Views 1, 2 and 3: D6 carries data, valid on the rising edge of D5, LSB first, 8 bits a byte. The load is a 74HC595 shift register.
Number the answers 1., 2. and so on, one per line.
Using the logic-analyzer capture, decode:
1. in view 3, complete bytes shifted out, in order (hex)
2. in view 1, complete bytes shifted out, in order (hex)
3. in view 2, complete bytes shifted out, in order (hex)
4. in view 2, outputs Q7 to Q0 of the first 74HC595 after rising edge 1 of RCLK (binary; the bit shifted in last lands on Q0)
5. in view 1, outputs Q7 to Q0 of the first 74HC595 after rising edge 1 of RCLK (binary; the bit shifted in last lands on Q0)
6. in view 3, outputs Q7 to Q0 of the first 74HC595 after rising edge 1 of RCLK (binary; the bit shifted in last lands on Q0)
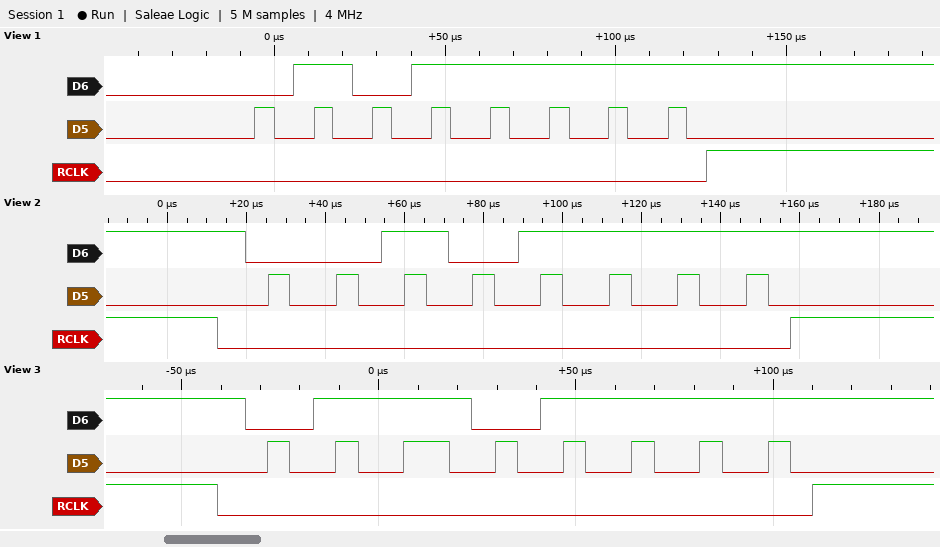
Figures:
1. F6
2. FA
3. F4
4. 00101111
5. 01011111
6. 01101111
